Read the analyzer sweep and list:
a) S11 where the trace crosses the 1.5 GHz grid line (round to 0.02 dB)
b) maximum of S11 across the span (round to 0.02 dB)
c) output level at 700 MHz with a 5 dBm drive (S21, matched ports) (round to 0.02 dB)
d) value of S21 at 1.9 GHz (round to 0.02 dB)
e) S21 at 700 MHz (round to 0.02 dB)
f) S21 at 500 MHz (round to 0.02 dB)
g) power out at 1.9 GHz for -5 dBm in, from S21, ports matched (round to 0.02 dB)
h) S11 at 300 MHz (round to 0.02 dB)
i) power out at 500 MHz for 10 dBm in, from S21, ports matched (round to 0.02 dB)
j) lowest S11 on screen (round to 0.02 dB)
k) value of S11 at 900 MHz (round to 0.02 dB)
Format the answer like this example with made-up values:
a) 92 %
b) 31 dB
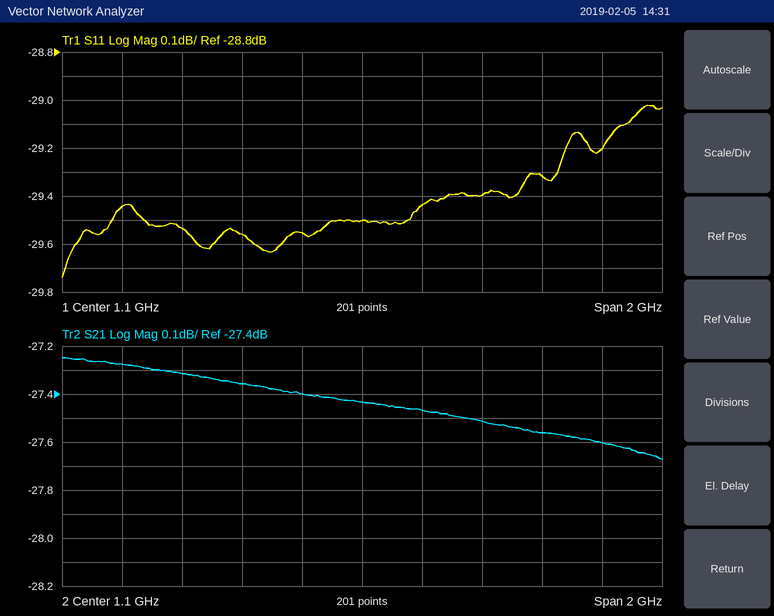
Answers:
a) -29.40 dB
b) -29.02 dB
c) -22.36 dBm
d) -27.60 dB
e) -27.36 dB
f) -27.32 dB
g) -32.60 dBm
h) -29.44 dB
i) -17.32 dBm
j) -29.74 dB
k) -29.56 dB
